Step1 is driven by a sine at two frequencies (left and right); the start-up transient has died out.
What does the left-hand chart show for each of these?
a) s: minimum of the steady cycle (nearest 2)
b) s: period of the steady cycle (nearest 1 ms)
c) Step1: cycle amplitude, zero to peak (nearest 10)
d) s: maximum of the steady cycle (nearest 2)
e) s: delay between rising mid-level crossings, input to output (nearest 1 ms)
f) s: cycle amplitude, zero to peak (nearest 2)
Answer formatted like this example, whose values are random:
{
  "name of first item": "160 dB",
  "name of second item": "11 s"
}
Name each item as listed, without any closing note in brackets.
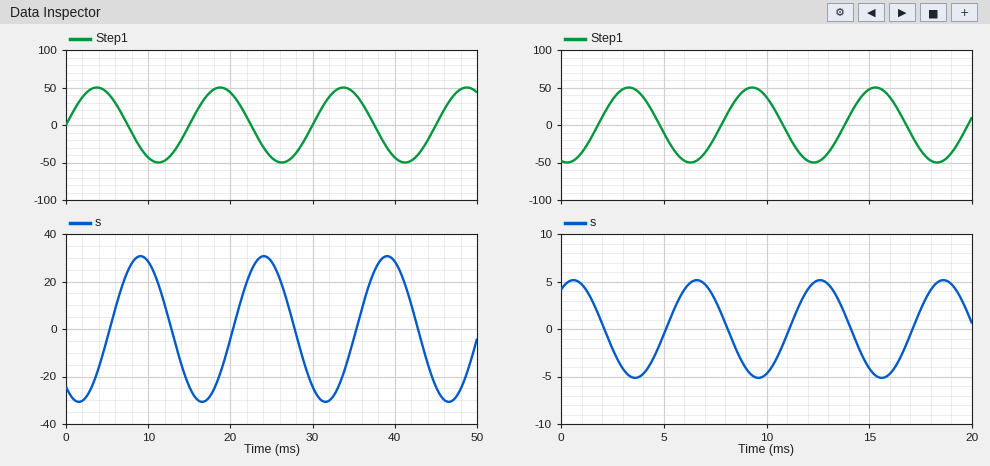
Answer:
{
  "s: minimum of the steady cycle": "-30",
  "s: period of the steady cycle": "15 ms",
  "Step1: cycle amplitude, zero to peak": "50",
  "s: maximum of the steady cycle": "30",
  "s: delay between rising mid-level crossings, input to output": "5 ms",
  "s: cycle amplitude, zero to peak": "30"
}
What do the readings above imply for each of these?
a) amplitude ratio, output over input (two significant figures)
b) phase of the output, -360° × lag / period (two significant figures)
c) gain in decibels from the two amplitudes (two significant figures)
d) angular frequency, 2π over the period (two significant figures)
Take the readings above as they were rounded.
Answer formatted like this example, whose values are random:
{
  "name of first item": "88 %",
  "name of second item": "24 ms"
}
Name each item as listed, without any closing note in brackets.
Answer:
{
  "amplitude ratio, output over input": "0.60",
  "phase of the output, -360° × lag / period": "-120°",
  "gain in decibels from the two amplitudes": "-4.4 dB",
  "angular frequency, 2π over the period": "0.42 rad/ms"
}
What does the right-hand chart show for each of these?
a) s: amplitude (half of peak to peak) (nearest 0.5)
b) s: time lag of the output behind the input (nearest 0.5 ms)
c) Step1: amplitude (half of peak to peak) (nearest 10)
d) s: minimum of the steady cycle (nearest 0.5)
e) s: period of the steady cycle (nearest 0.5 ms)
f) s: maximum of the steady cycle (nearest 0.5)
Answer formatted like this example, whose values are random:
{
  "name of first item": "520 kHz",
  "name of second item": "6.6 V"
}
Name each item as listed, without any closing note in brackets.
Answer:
{
  "s: amplitude (half of peak to peak)": "5.0",
  "s: time lag of the output behind the input": "3.5 ms",
  "Step1: amplitude (half of peak to peak)": "50",
  "s: minimum of the steady cycle": "-5.0",
  "s: period of the steady cycle": "6.0 ms",
  "s: maximum of the steady cycle": "5.0"
}
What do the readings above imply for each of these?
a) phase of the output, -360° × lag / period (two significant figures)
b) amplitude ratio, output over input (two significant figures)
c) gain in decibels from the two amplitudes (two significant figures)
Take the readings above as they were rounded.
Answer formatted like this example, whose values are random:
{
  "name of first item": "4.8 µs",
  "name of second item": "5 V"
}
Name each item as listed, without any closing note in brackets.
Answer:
{
  "phase of the output, -360° × lag / period": "-210°",
  "amplitude ratio, output over input": "0.10",
  "gain in decibels from the two amplitudes": "-20 dB"
}
